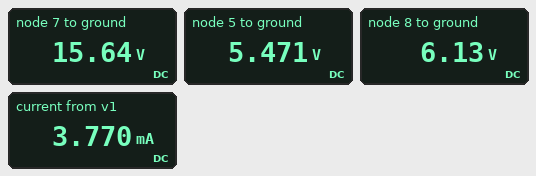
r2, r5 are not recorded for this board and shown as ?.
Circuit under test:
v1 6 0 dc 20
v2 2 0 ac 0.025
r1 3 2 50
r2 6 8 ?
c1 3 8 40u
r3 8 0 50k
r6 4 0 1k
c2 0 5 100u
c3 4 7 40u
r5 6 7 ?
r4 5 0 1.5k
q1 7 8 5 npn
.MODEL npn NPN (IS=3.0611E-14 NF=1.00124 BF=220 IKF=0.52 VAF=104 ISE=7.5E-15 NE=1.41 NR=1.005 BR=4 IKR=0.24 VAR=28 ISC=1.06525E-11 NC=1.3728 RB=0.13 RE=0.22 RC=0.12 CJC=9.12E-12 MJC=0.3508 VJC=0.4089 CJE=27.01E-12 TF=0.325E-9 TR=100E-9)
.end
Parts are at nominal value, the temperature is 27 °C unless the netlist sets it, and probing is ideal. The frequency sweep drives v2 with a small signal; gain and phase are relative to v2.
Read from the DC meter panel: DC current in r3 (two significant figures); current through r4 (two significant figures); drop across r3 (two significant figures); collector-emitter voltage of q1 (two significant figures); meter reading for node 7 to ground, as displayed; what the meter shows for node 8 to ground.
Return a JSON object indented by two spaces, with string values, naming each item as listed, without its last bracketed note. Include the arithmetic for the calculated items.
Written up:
{
  "DC current in r3": "(6.13 V) / 50 kΩ = 120 µA",
  "current through r4": "(5.471 V) / 1.5 kΩ = 3.6 mA",
  "drop across r3": "6.13 V = 6.1 V",
  "collector-emitter voltage of q1": "15.64 V - 5.471 V = 10 V",
  "meter reading for node 7 to ground, as displayed": "15.64 V",
  "what the meter shows for node 8 to ground": "6.13 V"
}
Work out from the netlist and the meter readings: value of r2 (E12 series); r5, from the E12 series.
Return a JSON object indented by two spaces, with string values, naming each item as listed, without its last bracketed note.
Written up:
{
  "value of r2": "100 kΩ",
  "r5, from the E12 series": "1.2 kΩ"
}
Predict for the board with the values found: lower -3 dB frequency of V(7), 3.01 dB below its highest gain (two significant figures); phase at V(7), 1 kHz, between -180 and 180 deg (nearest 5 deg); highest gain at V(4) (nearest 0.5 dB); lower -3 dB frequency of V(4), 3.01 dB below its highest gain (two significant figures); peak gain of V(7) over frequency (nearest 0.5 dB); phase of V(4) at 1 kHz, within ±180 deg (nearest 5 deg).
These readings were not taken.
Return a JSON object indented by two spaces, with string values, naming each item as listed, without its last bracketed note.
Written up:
{
  "lower -3 dB frequency of V(7), 3.01 dB below its highest gain": "210 Hz",
  "phase at V(7), 1 kHz, between -180 and 180 deg": "-170 deg",
  "highest gain at V(4)": "37.0 dB",
  "lower -3 dB frequency of V(4), 3.01 dB below its highest gain": "210 Hz",
  "peak gain of V(7) over frequency": "37.0 dB",
  "phase of V(4) at 1 kHz, within ±180 deg": "-170 deg"
}
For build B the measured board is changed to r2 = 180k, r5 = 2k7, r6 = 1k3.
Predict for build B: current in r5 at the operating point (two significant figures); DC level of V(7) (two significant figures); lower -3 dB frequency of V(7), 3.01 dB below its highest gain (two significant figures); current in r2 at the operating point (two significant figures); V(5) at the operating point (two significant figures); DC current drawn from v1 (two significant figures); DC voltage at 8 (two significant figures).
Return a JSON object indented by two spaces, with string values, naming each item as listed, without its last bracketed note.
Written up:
{
  "current in r5 at the operating point": "2.2 mA",
  "DC level of V(7)": "14 V",
  "lower -3 dB frequency of V(7), 3.01 dB below its highest gain": "130 Hz",
  "current in r2 at the operating point": "89 µA",
  "V(5) at the operating point": "3.3 V",
  "DC current drawn from v1": "2.3 mA",
  "DC voltage at 8": "4.0 V"
}
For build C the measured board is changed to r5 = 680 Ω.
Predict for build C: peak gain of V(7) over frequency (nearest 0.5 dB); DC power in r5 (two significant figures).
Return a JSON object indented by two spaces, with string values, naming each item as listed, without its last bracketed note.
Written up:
{
  "peak gain of V(7) over frequency": "34.5 dB",
  "DC power in r5": "9.0 mW"
}
